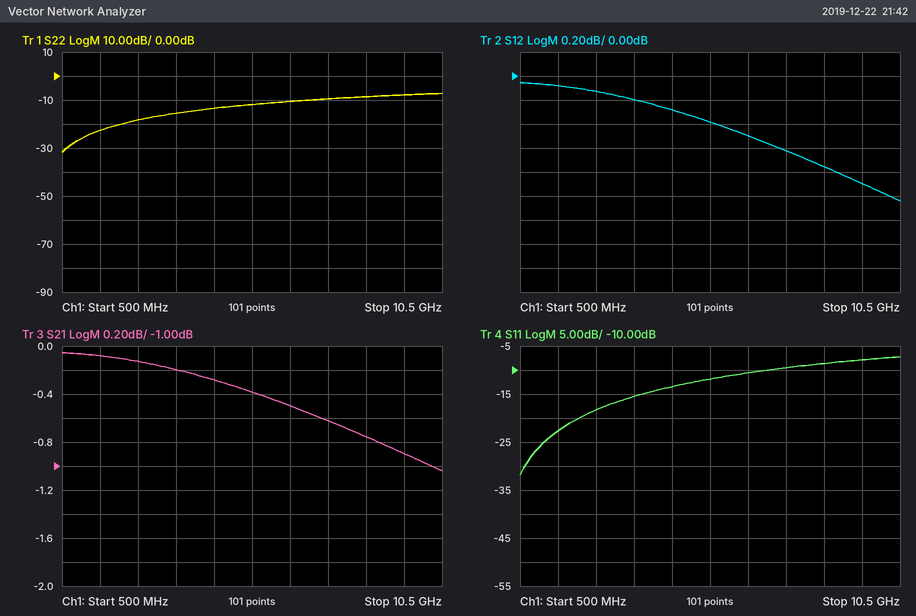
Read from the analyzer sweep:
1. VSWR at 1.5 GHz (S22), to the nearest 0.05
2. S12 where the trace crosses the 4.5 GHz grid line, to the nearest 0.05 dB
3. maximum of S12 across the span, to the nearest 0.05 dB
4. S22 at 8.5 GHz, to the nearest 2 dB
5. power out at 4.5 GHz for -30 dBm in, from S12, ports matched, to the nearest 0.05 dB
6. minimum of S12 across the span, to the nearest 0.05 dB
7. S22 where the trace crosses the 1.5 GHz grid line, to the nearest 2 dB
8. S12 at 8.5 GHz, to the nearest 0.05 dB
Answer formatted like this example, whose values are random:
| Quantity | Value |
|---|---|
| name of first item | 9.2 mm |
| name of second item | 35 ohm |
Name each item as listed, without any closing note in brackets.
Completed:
| Quantity | Value |
|---|---|
| VSWR at 1.5 GHz (S22), to the nearest 0.05 | 1.15 |
| S12 where the trace crosses the 4.5 GHz grid line, to the nearest 0.05 dB | -0.30 dB |
| maximum of S12 across the span, to the nearest 0.05 dB | -0.05 dB |
| S22 at 8.5 GHz, to the nearest 2 dB | -8 dB |
| power out at 4.5 GHz for -30 dBm in, from S12, ports matched, to the nearest 0.05 dB | -30.30 dBm |
| minimum of S12 across the span, to the nearest 0.05 dB | -1.05 dB |
| S22 where the trace crosses the 1.5 GHz grid line, to the nearest 2 dB | -22 dB |
| S12 at 8.5 GHz, to the nearest 0.05 dB | -0.75 dB |
